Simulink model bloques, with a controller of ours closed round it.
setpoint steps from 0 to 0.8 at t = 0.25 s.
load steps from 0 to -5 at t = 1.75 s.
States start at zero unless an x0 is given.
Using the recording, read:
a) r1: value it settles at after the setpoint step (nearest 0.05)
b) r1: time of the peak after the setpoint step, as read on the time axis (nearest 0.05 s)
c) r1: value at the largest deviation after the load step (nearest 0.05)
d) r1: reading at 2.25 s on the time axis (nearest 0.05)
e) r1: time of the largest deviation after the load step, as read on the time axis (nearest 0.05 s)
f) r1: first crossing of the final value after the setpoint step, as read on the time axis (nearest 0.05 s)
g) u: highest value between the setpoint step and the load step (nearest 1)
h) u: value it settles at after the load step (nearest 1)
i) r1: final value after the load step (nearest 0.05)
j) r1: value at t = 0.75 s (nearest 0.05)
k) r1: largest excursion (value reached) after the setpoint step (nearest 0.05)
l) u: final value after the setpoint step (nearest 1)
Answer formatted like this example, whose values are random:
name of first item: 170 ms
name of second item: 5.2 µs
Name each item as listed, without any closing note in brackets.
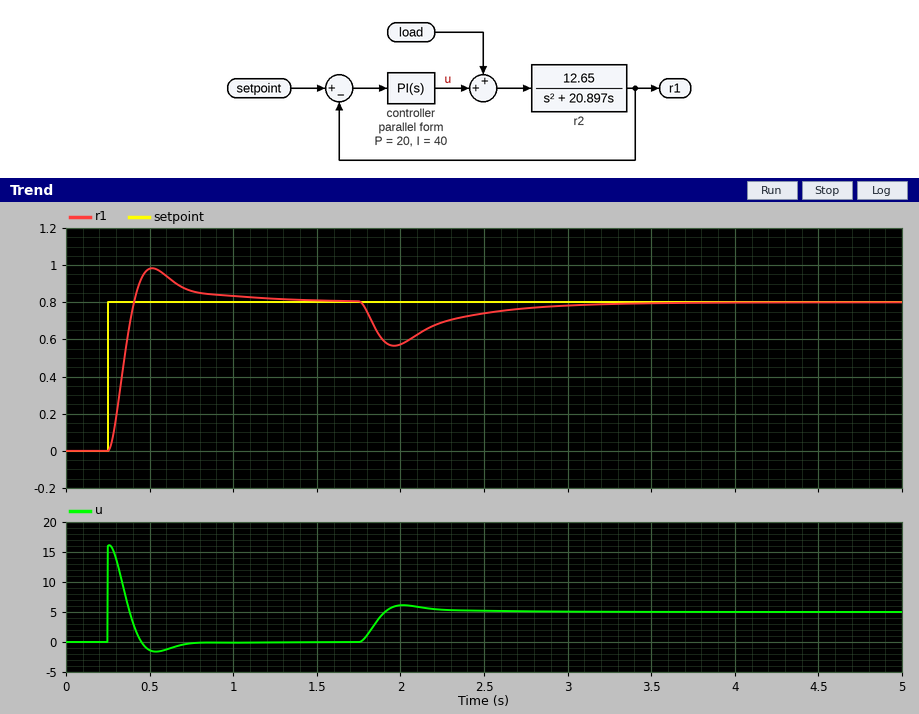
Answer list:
r1: value it settles at after the setpoint step: 0.80
r1: time of the peak after the setpoint step, as read on the time axis: 0.50 s
r1: value at the largest deviation after the load step: 0.55
r1: reading at 2.25 s on the time axis: 0.70
r1: time of the largest deviation after the load step, as read on the time axis: 1.95 s
r1: first crossing of the final value after the setpoint step, as read on the time axis: 0.40 s
u: highest value between the setpoint step and the load step: 16
u: value it settles at after the load step: 5
r1: final value after the load step: 0.80
r1: value at t = 0.75 s: 0.85
r1: largest excursion (value reached) after the setpoint step: 1.00
u: final value after the setpoint step: 0
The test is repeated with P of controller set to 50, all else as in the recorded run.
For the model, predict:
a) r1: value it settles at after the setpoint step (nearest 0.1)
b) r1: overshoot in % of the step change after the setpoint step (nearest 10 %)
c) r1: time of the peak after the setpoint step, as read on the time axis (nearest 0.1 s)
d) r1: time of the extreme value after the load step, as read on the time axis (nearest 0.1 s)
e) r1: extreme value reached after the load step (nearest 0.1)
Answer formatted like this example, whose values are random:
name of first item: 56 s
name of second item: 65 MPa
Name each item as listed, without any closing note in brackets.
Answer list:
r1: value it settles at after the setpoint step: 0.8
r1: overshoot in % of the step change after the setpoint step: 30 %
r1: time of the peak after the setpoint step, as read on the time axis: 0.4 s
r1: time of the extreme value after the load step, as read on the time axis: 1.9 s
r1: extreme value reached after the load step: 0.7
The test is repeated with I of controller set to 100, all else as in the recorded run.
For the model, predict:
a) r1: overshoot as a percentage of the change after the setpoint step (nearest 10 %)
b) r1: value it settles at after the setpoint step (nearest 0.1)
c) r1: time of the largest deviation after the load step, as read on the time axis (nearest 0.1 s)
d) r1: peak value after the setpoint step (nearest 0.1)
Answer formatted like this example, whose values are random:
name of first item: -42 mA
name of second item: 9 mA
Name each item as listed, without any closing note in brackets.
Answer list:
r1: overshoot as a percentage of the change after the setpoint step: 40 %
r1: value it settles at after the setpoint step: 0.8
r1: time of the largest deviation after the load step, as read on the time axis: 1.9 s
r1: peak value after the setpoint step: 1.1
